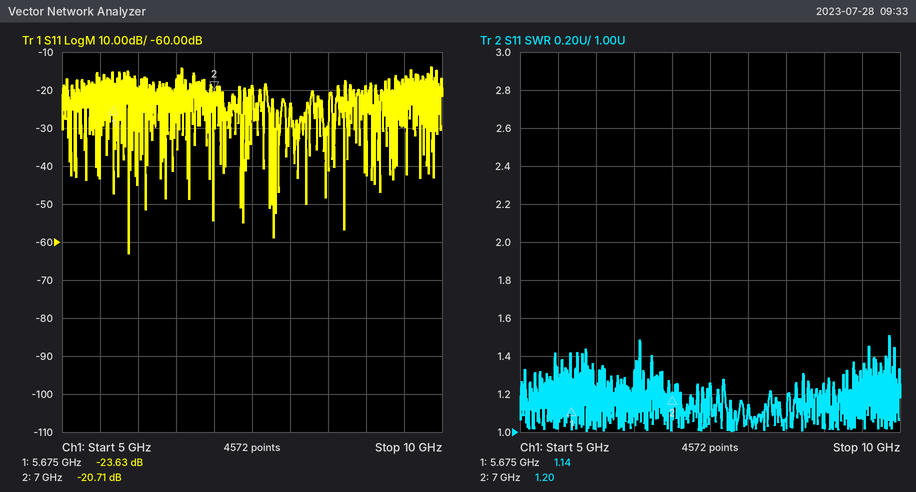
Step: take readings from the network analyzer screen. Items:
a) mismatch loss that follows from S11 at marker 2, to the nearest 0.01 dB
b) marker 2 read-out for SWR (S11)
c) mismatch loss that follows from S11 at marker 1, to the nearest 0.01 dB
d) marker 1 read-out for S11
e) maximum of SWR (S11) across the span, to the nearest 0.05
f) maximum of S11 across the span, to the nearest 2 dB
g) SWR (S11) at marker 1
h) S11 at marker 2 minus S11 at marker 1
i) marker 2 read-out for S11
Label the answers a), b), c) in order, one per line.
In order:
a) 0.04 dB
b) 1.20
c) 0.02 dB
d) -23.63 dB
e) 1.50
f) -14 dB
g) 1.14
h) 2.92 dB
i) -20.71 dB
